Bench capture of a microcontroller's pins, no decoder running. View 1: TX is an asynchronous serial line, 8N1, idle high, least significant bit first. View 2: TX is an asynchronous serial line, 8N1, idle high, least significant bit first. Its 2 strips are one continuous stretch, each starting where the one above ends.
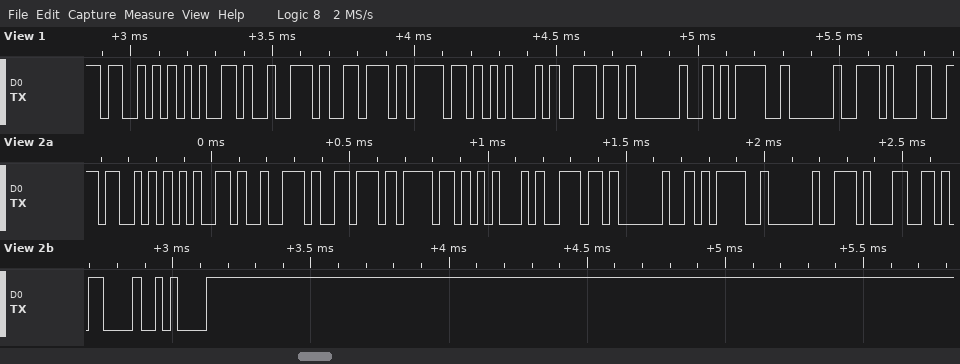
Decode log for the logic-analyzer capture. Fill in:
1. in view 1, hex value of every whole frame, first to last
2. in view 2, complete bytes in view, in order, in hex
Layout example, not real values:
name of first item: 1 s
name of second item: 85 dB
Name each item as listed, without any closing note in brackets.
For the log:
in view 1, hex value of every whole frame, first to last: 0x53 0x65 0x72 0x76 0x6F 0x45 0x6E 0x20 0x3D 0x20 0x31
in view 2, complete bytes in view, in order, in hex: 53 65 72 76 6F 45 6E 20 3D 20 31 0D 0A
